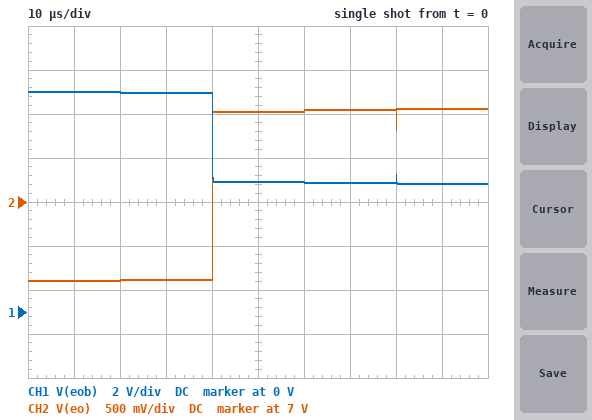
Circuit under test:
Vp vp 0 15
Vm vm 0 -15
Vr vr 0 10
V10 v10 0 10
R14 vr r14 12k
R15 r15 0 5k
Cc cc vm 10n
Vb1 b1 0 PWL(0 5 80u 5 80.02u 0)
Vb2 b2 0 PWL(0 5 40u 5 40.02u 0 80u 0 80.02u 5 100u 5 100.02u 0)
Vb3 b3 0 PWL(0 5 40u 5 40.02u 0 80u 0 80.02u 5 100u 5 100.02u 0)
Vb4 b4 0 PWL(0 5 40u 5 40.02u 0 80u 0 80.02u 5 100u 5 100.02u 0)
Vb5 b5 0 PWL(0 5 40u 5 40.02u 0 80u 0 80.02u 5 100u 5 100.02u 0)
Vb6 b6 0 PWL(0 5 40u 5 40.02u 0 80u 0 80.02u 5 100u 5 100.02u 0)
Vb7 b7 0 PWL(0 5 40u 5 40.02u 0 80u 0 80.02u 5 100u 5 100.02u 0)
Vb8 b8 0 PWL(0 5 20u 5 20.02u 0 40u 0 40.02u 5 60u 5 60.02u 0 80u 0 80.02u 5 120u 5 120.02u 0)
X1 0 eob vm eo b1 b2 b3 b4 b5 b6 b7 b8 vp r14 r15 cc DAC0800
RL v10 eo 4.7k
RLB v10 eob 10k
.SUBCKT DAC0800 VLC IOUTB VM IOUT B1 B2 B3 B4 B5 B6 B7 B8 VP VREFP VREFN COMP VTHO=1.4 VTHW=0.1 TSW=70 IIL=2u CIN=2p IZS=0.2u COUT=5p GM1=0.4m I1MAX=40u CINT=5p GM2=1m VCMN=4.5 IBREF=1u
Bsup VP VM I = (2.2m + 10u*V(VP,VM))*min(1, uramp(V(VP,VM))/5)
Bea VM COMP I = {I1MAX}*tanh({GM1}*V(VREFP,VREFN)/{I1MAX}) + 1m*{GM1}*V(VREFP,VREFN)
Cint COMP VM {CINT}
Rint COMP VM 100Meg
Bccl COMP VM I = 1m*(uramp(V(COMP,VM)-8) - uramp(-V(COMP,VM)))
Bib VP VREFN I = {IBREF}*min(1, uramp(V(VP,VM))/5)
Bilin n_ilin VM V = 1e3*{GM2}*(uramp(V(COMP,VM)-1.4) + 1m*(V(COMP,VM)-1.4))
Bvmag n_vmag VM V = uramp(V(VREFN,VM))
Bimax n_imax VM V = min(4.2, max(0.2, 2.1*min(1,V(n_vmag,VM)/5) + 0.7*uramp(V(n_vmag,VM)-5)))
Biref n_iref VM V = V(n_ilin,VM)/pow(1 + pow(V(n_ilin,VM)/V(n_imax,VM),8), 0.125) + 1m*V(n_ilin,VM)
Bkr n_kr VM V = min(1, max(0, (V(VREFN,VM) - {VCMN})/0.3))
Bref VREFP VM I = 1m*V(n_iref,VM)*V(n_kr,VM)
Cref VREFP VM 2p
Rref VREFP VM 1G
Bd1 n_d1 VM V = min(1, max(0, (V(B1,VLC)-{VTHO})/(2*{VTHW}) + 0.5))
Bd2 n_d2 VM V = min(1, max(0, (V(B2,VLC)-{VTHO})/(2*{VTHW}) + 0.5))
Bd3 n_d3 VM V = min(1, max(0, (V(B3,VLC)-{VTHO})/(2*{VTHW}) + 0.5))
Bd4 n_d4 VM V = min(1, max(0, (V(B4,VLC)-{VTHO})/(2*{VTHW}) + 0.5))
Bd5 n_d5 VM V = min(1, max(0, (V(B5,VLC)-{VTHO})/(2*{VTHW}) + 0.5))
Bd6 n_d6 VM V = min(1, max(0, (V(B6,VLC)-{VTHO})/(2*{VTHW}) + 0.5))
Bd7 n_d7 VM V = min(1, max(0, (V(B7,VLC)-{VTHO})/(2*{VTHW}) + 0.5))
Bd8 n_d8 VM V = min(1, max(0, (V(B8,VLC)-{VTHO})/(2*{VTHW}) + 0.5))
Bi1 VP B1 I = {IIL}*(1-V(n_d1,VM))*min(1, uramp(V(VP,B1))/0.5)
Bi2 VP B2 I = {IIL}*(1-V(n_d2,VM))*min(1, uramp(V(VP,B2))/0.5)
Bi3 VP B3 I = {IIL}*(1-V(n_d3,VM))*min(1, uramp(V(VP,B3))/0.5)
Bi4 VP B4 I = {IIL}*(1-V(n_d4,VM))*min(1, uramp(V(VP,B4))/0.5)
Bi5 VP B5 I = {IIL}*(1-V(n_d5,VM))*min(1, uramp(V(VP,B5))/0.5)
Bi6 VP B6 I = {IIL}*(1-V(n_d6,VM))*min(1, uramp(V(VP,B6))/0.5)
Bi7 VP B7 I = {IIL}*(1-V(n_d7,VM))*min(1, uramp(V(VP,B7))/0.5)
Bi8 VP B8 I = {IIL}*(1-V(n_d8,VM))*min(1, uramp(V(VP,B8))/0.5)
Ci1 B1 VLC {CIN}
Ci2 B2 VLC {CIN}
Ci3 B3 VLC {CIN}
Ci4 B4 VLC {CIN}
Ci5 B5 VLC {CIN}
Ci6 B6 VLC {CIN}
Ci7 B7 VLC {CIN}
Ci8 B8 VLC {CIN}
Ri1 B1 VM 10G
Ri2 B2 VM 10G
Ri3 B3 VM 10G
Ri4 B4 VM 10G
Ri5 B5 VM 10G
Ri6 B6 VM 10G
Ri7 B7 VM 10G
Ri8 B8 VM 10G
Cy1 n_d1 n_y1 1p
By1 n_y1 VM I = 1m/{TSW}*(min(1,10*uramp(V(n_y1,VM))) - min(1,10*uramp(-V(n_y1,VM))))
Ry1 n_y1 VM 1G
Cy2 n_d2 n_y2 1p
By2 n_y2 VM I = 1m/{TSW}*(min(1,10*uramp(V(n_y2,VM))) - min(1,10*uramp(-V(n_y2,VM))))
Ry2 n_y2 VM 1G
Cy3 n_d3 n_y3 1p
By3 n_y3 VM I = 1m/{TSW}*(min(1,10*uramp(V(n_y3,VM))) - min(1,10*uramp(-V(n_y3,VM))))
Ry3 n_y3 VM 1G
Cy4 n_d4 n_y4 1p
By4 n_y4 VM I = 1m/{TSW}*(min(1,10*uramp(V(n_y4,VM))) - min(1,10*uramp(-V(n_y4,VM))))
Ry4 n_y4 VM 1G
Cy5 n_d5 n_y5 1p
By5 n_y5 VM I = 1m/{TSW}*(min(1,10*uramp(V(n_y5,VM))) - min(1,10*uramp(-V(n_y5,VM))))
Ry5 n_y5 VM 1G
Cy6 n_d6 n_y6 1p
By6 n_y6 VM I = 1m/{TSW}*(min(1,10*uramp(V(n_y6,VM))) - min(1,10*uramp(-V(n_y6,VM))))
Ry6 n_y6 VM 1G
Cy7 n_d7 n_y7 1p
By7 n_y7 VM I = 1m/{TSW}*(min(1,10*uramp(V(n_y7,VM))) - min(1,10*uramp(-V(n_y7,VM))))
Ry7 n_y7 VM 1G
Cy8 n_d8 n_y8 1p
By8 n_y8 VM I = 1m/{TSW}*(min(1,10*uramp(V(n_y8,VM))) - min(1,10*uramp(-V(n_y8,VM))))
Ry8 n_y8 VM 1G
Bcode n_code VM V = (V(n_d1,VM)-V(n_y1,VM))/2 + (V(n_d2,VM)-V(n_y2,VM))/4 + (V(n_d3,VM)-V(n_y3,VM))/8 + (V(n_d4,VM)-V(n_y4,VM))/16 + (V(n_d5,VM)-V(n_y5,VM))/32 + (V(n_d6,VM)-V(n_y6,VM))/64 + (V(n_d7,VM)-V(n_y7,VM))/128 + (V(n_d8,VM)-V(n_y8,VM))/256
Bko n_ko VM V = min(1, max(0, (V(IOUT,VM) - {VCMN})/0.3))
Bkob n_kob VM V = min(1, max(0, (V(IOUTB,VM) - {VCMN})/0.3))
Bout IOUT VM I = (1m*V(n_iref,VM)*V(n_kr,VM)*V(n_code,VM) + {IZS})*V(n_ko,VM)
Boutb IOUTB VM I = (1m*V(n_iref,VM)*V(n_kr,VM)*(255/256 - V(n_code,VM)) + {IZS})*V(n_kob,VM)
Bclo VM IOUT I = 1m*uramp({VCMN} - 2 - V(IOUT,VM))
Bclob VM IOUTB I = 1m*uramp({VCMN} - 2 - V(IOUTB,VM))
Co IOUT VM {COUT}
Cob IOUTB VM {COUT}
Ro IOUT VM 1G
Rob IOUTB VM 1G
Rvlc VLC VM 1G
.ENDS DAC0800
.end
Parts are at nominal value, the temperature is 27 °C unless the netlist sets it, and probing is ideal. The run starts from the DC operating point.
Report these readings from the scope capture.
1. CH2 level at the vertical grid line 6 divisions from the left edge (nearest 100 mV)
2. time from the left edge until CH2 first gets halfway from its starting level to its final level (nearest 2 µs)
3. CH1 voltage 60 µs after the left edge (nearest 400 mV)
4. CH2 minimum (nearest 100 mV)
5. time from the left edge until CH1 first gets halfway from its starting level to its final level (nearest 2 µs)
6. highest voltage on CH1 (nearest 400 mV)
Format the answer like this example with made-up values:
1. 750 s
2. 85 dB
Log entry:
1. 8.0 V
2. 40 µs
3. 6.0 V
4. 6.1 V
5. 40 µs
6. 10.0 V
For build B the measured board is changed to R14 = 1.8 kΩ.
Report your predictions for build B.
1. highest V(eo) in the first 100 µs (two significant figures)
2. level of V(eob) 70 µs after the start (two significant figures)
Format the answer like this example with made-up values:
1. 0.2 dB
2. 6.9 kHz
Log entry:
1. 220 mV
2. -10 V
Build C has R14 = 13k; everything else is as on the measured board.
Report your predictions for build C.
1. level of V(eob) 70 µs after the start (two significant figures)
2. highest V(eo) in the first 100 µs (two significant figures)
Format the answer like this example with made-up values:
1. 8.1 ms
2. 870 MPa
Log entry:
1. 6.2 V
2. 8.2 V
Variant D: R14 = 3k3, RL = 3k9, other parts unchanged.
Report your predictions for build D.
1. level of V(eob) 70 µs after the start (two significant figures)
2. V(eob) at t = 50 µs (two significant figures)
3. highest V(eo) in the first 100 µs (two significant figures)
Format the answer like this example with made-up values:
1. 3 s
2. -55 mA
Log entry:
1. -5.0 V
2. -4.9 V
3. 4.1 V
